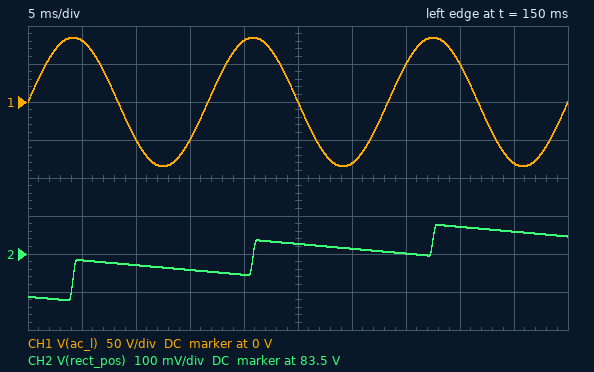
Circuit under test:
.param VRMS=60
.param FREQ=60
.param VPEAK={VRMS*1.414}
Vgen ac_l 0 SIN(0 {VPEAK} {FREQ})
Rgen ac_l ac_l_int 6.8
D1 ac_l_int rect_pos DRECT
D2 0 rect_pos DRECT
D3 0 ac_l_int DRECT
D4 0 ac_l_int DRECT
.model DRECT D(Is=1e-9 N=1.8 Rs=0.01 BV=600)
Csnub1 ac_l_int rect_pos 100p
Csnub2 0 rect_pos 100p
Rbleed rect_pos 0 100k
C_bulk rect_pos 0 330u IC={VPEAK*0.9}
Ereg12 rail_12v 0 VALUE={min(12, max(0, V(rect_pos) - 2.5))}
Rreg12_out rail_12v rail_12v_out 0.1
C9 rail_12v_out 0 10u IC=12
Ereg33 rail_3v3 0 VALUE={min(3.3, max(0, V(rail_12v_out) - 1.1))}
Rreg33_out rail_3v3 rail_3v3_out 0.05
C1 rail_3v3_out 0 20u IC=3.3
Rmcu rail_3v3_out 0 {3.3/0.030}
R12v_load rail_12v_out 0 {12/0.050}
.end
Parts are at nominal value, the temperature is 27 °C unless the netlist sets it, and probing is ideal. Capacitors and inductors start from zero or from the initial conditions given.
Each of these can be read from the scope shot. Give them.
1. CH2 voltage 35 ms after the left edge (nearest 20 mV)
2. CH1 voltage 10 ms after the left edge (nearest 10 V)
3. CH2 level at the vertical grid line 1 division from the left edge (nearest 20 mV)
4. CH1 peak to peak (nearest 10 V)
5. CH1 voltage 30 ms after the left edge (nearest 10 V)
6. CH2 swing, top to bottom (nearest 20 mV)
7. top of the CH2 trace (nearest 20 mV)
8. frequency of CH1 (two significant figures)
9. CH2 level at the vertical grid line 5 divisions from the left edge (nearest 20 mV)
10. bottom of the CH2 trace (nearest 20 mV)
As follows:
83.50 V
-50 V
83.48 V
170 V
-80 V
200 mV
83.58 V
60 Hz
83.52 V
83.38 V
